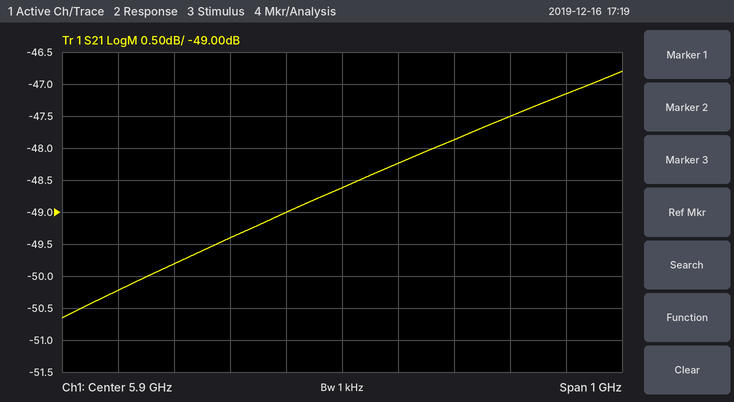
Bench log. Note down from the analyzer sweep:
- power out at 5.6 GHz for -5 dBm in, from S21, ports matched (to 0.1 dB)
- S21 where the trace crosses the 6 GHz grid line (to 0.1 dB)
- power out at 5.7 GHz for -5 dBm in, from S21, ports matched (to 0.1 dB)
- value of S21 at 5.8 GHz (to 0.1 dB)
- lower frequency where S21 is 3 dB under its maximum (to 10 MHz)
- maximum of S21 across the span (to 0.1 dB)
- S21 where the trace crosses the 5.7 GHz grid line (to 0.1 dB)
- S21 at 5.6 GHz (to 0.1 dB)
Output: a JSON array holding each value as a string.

["-54.8 dBm", "-48.2 dB", "-54.4 dBm", "-49.0 dB", "5.60 GHz", "-46.8 dB", "-49.4 dB", "-49.8 dB"]
